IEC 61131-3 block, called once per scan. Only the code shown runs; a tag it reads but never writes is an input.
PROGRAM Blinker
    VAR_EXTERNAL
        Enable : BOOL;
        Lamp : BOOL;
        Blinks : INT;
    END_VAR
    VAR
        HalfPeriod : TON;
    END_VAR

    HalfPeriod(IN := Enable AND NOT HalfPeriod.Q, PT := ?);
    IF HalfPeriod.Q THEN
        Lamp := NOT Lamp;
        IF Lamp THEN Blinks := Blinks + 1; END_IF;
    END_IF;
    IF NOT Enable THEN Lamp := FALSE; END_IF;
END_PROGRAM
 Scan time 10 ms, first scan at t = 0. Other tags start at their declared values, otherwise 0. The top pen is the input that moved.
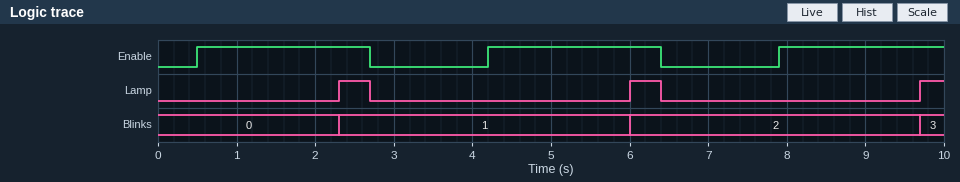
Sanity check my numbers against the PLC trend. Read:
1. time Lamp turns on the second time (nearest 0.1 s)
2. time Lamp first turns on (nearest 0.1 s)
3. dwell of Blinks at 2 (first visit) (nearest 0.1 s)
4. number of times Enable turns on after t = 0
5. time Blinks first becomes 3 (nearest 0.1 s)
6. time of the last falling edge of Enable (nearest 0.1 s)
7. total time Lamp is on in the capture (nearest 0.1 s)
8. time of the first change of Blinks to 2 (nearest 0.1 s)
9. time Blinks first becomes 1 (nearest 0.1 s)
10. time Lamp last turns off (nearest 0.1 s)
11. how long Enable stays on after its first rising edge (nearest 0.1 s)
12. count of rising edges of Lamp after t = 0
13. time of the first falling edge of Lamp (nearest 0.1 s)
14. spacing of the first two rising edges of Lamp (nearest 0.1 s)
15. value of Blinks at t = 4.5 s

6.0 s
2.3 s
3.7 s
3
9.7 s
6.4 s
1.1 s
6.0 s
2.3 s
6.4 s
2.2 s
3
2.7 s
3.7 s
1
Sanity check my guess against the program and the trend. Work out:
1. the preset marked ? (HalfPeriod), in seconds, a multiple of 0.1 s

1.8 s
